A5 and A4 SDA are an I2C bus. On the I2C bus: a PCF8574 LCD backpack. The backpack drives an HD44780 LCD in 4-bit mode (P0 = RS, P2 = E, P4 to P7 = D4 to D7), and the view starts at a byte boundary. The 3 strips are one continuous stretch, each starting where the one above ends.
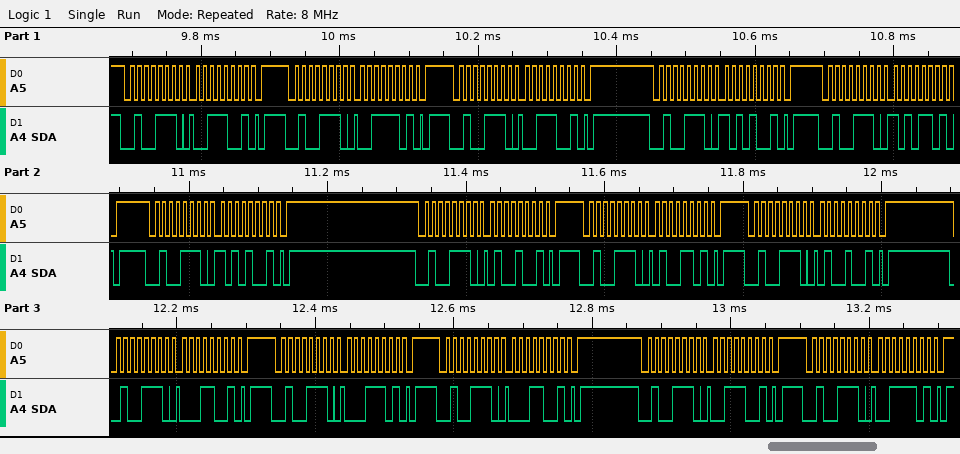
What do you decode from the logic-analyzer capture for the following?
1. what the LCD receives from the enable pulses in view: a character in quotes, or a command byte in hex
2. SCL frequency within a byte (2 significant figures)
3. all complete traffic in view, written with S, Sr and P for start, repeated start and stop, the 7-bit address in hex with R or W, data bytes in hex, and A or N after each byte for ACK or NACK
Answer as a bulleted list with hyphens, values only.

- ':' 'A'
- 100 kHz
- S 27W A 39 A P S 27W A 3D A P S 27W A 39 A P S 27W A A9 A P S 27W A AD A P S 27W A A9 A P S 27W A 49 A P S 27W A 4D A P S 27W A 49 A P S 27W A 19 A P S 27W A 1D A P S 27W A 19 A P S 27W A 39 A P S 27W A 3D A P
